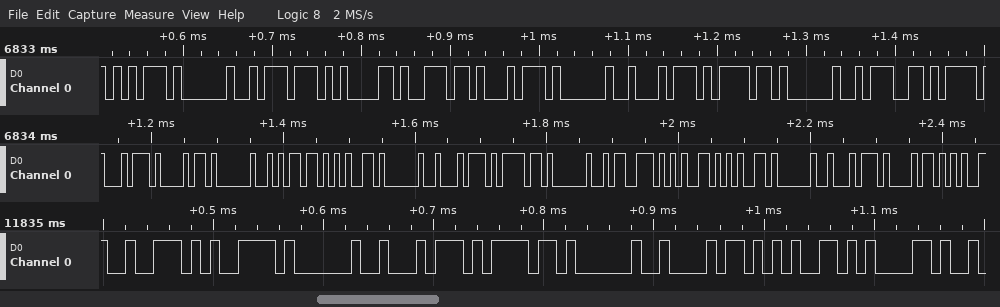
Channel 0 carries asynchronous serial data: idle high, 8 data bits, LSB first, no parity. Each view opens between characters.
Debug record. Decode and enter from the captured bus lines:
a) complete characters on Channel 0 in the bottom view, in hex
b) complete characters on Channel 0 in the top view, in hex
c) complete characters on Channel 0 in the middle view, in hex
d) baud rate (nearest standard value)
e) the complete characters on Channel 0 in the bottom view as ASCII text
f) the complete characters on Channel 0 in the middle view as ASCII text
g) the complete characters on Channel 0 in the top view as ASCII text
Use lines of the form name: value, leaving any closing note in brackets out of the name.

complete characters on Channel 0 in the bottom view, in hex: 72, 79, 20, 74, 6F, 20, 68, 65, 61
complete characters on Channel 0 in the top view, in hex: 75, 20, 77, 61, 6E, 74, 20, 74, 6F, 20, 67
complete characters on Channel 0 in the middle view, in hex: 74, 68, 20, 6D, 65, 20, 74, 6F, 20, 73, 65, 65, 20, 74, 68
baud rate: 115200 baud
the complete characters on Channel 0 in the bottom view as ASCII text: "ry to hea"
the complete characters on Channel 0 in the middle view as ASCII text: "th me to see th"
the complete characters on Channel 0 in the top view as ASCII text: "u want to g"
